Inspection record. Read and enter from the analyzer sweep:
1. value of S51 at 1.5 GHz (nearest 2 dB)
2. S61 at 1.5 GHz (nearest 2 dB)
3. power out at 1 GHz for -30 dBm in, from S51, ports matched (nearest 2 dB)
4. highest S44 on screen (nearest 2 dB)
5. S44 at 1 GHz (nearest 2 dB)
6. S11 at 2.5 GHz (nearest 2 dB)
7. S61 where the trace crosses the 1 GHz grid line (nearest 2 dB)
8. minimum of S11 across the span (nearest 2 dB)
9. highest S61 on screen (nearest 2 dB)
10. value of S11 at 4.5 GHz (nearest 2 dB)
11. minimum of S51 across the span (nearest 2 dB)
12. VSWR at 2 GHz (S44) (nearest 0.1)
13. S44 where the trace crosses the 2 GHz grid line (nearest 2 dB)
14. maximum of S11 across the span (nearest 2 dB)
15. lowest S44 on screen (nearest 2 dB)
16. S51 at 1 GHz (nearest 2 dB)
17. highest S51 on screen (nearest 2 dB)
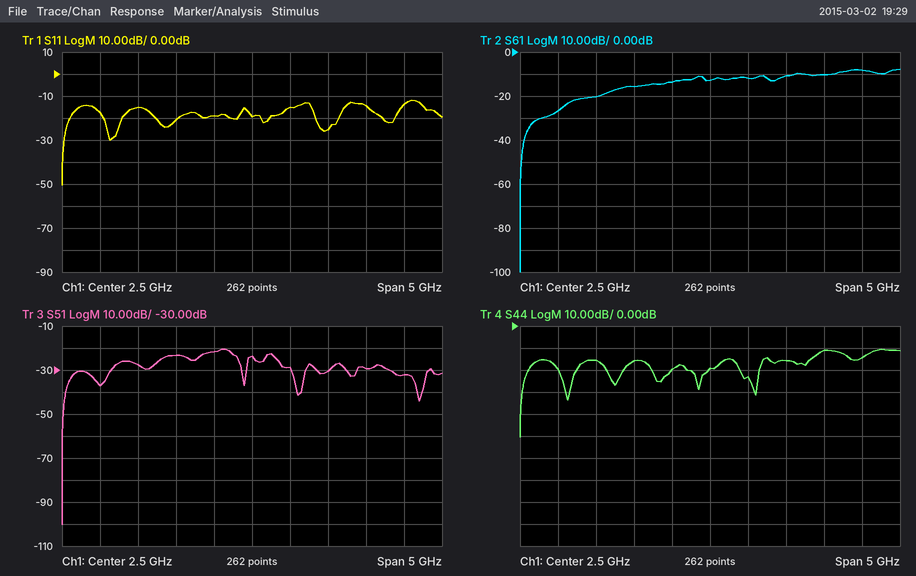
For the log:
-24 dB
-16 dB
-58 dBm
-10 dB
-16 dB
-20 dB
-20 dB
-50 dB
-8 dB
-14 dB
-100 dB
1.2
-20 dB
-12 dB
-50 dB
-28 dB
-20 dB
